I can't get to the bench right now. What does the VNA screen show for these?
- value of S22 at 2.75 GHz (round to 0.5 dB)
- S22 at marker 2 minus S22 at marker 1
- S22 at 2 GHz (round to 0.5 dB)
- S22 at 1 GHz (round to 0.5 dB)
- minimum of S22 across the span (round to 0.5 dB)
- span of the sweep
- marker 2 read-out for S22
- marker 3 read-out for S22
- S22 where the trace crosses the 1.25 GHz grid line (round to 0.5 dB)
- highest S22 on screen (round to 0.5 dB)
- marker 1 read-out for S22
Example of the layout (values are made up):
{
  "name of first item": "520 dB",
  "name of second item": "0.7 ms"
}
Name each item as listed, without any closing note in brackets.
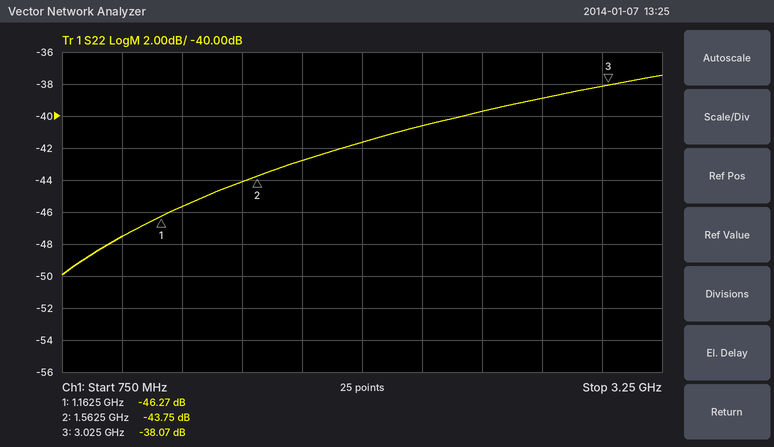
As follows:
{
  "value of S22 at 2.75 GHz": "-39.0 dB",
  "S22 at marker 2 minus S22 at marker 1": "2.52 dB",
  "S22 at 2 GHz": "-41.5 dB",
  "S22 at 1 GHz": "-47.5 dB",
  "minimum of S22 across the span": "-50.0 dB",
  "span of the sweep": "2.5 GHz",
  "marker 2 read-out for S22": "-43.75 dB",
  "marker 3 read-out for S22": "-38.07 dB",
  "S22 where the trace crosses the 1.25 GHz grid line": "-45.5 dB",
  "highest S22 on screen": "-37.5 dB",
  "marker 1 read-out for S22": "-46.27 dB"
}
